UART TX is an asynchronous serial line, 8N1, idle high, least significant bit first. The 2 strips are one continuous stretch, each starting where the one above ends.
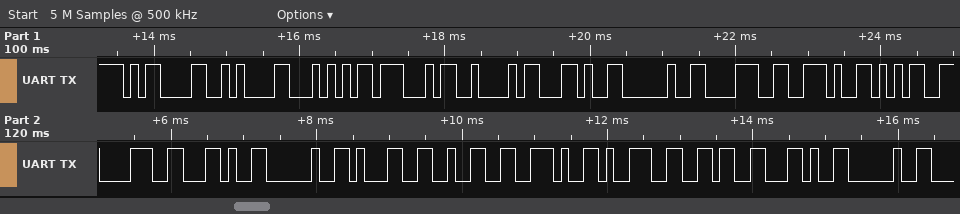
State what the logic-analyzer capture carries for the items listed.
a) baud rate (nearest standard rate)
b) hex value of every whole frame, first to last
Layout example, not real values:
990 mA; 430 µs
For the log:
9600 baud; 0x0D 0x0A 0x54 0x47 0x42 0x2C 0x20 0x38 0x2E 0x35 0x38 0x2C 0x20 0x31 0x32 0x2E 0x39 0x36 0x2C 0x20
